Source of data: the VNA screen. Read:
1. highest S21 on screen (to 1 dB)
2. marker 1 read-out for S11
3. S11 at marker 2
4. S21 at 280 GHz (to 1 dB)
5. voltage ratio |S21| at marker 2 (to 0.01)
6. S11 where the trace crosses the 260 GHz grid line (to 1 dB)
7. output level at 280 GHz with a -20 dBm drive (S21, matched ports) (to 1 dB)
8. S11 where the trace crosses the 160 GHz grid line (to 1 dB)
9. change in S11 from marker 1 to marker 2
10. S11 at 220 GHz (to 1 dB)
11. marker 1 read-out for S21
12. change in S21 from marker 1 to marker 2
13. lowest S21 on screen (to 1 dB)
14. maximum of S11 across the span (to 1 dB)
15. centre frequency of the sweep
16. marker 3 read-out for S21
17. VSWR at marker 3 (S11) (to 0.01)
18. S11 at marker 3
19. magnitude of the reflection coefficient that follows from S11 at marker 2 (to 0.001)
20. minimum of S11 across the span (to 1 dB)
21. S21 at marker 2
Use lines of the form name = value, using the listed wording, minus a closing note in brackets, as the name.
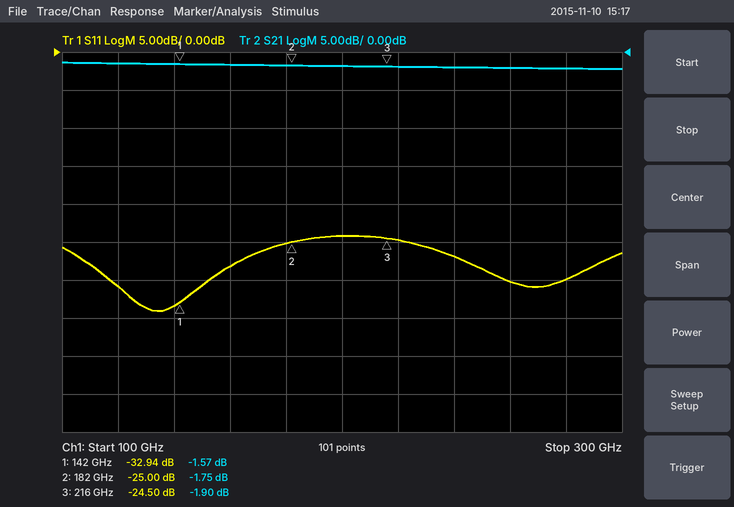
highest S21 on screen = -1 dB
marker 1 read-out for S11 = -32.94 dB
S11 at marker 2 = -25.00 dB
S21 at 280 GHz = -2 dB
voltage ratio |S21| at marker 2 = 0.82
S11 where the trace crosses the 260 GHz grid line = -30 dB
output level at 280 GHz with a -20 dBm drive (S21, matched ports) = -22 dBm
S11 where the trace crosses the 160 GHz grid line = -28 dB
change in S11 from marker 1 to marker 2 = 7.94 dB
S11 at 220 GHz = -25 dB
marker 1 read-out for S21 = -1.57 dB
change in S21 from marker 1 to marker 2 = -0.18 dB
lowest S21 on screen = -2 dB
maximum of S11 across the span = -24 dB
centre frequency of the sweep = 200 GHz
marker 3 read-out for S21 = -1.90 dB
VSWR at marker 3 (S11) = 1.13
S11 at marker 3 = -24.50 dB
magnitude of the reflection coefficient that follows from S11 at marker 2 = 0.056
minimum of S11 across the span = -34 dB
S21 at marker 2 = -1.75 dB
